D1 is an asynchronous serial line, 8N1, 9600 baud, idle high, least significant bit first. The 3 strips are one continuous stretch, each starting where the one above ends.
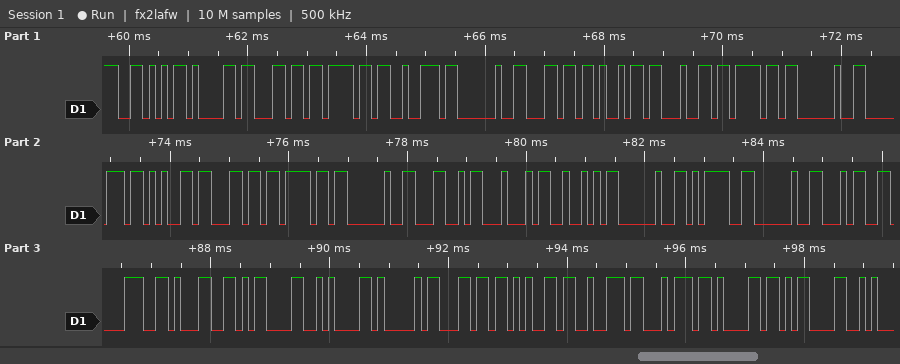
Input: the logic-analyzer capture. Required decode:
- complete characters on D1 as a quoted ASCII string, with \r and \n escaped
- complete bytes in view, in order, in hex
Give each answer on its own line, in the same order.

"Valor lido pelo LDR = 481\r\nAlerta\r"
0x56 0x61 0x6C 0x6F 0x72 0x20 0x6C 0x69 0x64 0x6F 0x20 0x70 0x65 0x6C 0x6F 0x20 0x4C 0x44 0x52 0x20 0x3D 0x20 0x34 0x38 0x31 0x0D 0x0A 0x41 0x6C 0x65 0x72 0x74 0x61 0x0D
